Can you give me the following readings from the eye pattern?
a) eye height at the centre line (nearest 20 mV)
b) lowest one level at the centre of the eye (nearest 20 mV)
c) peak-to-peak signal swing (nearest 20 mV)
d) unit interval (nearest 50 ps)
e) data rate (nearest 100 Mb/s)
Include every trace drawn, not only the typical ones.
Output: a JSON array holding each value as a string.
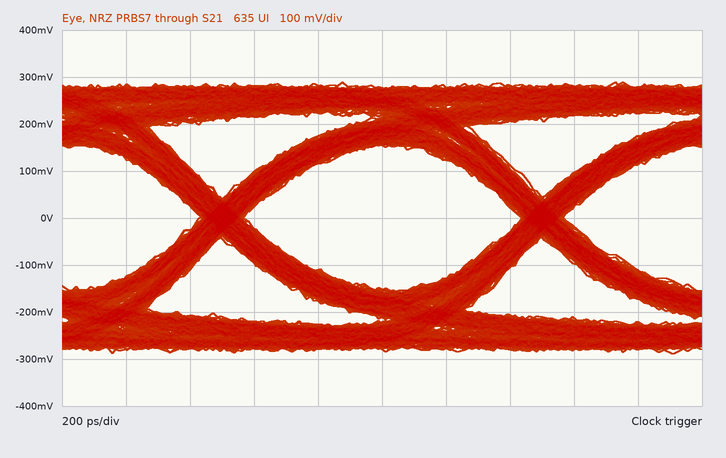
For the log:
["300 mV", "160 mV", "580 mV", "1.00 ns", "1.0 Gb/s"]
